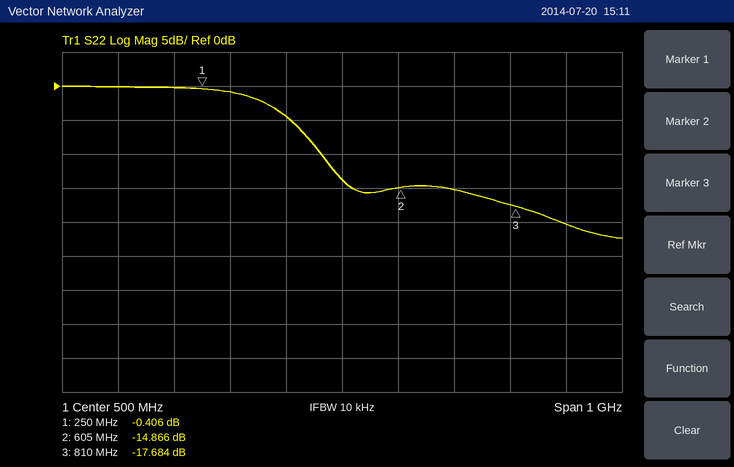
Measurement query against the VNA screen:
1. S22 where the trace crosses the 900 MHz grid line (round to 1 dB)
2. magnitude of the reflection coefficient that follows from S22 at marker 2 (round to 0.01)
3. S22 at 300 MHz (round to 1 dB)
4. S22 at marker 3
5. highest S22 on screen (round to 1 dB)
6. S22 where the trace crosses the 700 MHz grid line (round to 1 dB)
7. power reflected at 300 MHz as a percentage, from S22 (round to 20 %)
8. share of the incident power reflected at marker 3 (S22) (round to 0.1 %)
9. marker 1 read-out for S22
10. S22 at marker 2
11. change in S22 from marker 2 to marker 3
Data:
-20 dB
0.18
-1 dB
-17.684 dB
0 dB
-15 dB
80 %
1.7 %
-0.406 dB
-14.866 dB
-2.818 dB
